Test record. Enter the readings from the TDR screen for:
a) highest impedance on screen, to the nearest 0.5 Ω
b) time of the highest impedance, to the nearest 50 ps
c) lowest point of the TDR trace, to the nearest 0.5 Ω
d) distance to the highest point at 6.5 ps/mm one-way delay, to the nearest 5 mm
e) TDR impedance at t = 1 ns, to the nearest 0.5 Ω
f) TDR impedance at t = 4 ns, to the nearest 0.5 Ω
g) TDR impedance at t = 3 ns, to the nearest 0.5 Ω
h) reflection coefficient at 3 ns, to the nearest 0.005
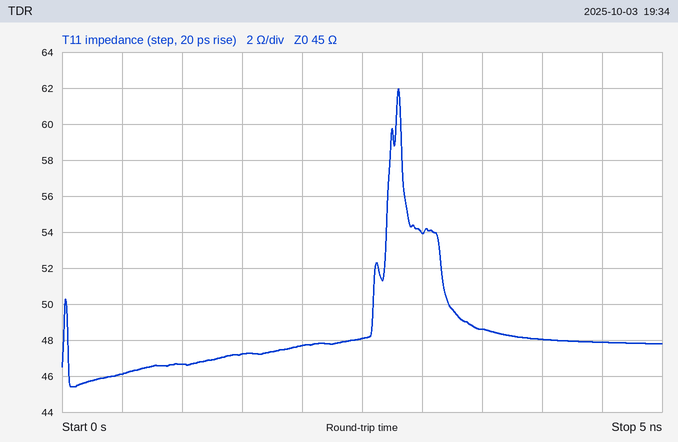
62.0 Ω
2.80 ns
45.5 Ω
215 mm
46.5 Ω
48.0 Ω
54.0 Ω
+0.090
